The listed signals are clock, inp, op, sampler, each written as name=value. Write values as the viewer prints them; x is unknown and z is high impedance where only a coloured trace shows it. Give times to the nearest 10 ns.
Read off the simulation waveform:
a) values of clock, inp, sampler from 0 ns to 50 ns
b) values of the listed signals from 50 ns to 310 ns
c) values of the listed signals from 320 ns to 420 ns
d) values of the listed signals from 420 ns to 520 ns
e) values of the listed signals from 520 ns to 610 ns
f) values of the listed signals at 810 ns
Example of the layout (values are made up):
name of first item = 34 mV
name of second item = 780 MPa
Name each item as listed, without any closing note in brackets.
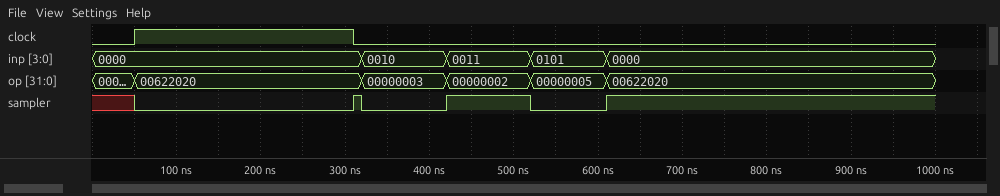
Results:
values of clock, inp, sampler from 0 ns to 50 ns = clock=0, inp=0000, sampler=x
values of the listed signals from 50 ns to 310 ns = clock=1, inp=0000, op=00622020, sampler=0
values of the listed signals from 320 ns to 420 ns = clock=0, inp=0010, op=00000003, sampler=0
values of the listed signals from 420 ns to 520 ns = clock=0, inp=0011, op=00000002, sampler=1
values of the listed signals from 520 ns to 610 ns = clock=0, inp=0101, op=00000005, sampler=0
values of the listed signals at 810 ns = clock=0, inp=0000, op=00622020, sampler=1
